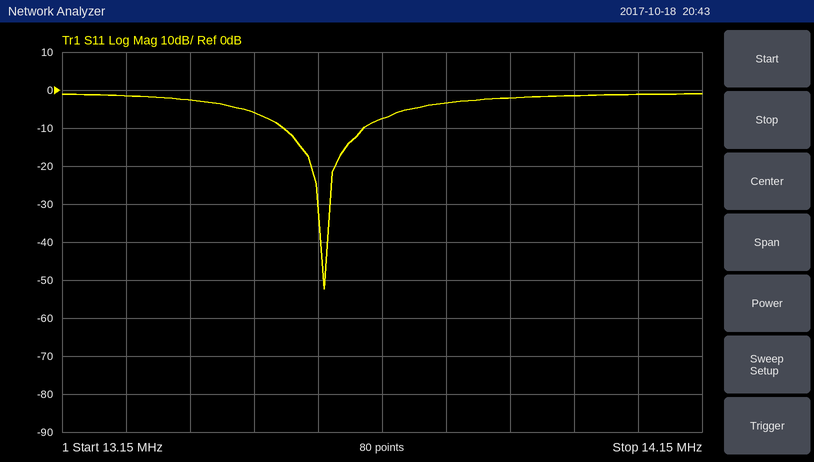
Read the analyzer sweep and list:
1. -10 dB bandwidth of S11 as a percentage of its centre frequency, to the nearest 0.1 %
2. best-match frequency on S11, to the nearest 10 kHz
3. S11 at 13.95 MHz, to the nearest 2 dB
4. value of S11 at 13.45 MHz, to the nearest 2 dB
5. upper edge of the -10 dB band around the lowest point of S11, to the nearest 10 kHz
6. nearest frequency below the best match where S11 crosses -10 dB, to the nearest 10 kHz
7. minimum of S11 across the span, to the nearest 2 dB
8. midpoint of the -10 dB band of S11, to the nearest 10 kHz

0.9 %
13.56 MHz
-2 dB
-6 dB
13.62 MHz
13.50 MHz
-52 dB
13.56 MHz
